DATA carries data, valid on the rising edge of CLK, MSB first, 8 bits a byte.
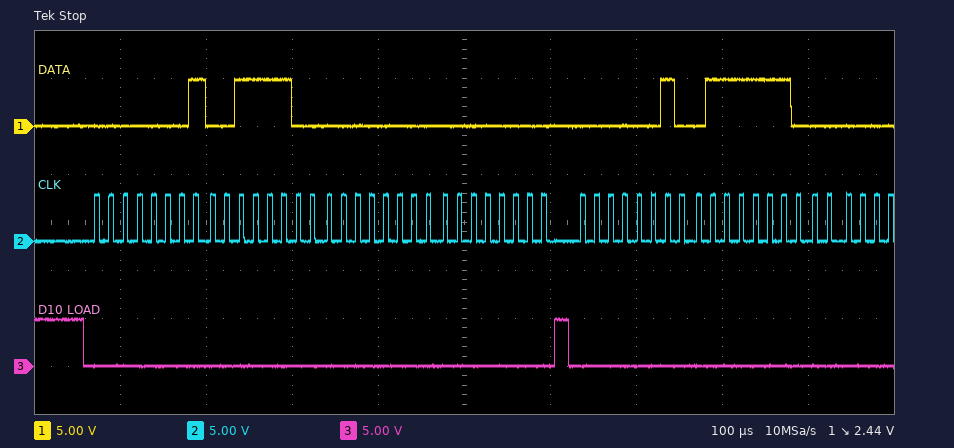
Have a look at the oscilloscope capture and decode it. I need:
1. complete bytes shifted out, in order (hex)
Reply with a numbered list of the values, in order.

1. 01 3C 00 00 02 7E
